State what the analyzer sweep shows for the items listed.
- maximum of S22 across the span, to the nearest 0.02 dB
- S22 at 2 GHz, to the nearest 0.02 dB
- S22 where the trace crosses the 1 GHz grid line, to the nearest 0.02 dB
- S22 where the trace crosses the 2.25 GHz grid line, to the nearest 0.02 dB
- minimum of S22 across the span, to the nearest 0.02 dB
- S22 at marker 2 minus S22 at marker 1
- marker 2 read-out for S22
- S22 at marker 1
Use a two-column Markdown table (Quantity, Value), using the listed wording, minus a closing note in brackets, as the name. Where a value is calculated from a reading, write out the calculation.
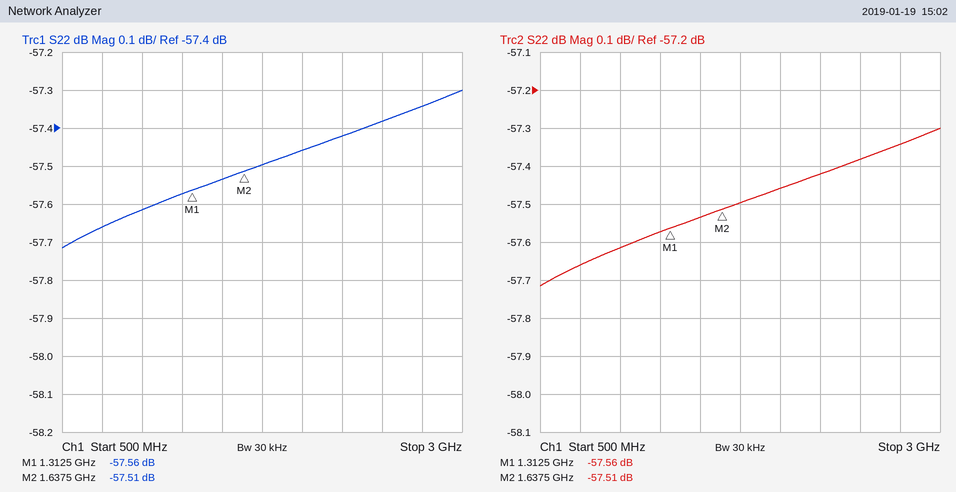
| Quantity | Value |
|---|---|
| maximum of S22 across the span, to the nearest 0.02 dB | -57.30 dB |
| S22 at 2 GHz, to the nearest 0.02 dB | -57.46 dB |
| S22 where the trace crosses the 1 GHz grid line, to the nearest 0.02 dB | -57.62 dB |
| S22 where the trace crosses the 2.25 GHz grid line, to the nearest 0.02 dB | -57.42 dB |
| minimum of S22 across the span, to the nearest 0.02 dB | -57.72 dB |
| S22 at marker 2 minus S22 at marker 1 | -57.51 − (-57.56) = 0.05 dB |
| marker 2 read-out for S22 | -57.51 dB |
| S22 at marker 1 | -57.56 dB |
